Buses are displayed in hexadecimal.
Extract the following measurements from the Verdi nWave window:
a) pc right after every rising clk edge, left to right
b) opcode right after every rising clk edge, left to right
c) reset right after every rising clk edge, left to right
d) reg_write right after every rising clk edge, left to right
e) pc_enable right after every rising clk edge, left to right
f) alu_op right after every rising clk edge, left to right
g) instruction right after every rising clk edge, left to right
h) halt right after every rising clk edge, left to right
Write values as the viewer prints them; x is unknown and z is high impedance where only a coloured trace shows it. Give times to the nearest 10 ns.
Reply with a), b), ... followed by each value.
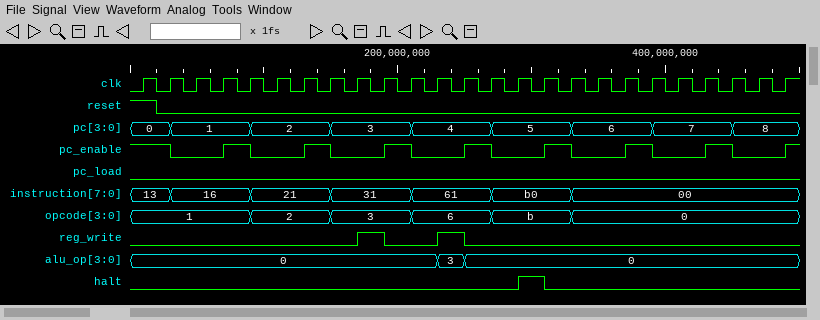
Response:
a) 0, 1, 1, 1, 2, 2, 2, 3, 3, 3, 4, 4, 4, 5, 5, 5, 6, 6, 6, 7, 7, 7, 8, 8, 8
b) 1, 1, 1, 1, 2, 2, 2, 3, 3, 3, 6, 6, 6, b, b, b, 0, 0, 0, 0, 0, 0, 0, 0, 0
c) 1 0 0 0 0 0 0 0 0 0 0 0 0 0 0 0 0 0 0 0 0 0 0 0 0
d) 0 0 0 0 0 0 0 0 1 0 0 1 0 0 0 0 0 0 0 0 0 0 0 0 0
e) 1 0 0 1 0 0 1 0 0 1 0 0 1 0 0 1 0 0 1 0 0 1 0 0 1
f) 0, 0, 0, 0, 0, 0, 0, 0, 0, 0, 0, 3, 0, 0, 0, 0, 0, 0, 0, 0, 0, 0, 0, 0, 0
g) 13, 16, 16, 16, 21, 21, 21, 31, 31, 31, 61, 61, 61, b0, b0, b0, 00, 00, 00, 00, 00, 00, 00, 00, 00
h) 0 0 0 0 0 0 0 0 0 0 0 0 0 0 1 0 0 0 0 0 0 0 0 0 0
